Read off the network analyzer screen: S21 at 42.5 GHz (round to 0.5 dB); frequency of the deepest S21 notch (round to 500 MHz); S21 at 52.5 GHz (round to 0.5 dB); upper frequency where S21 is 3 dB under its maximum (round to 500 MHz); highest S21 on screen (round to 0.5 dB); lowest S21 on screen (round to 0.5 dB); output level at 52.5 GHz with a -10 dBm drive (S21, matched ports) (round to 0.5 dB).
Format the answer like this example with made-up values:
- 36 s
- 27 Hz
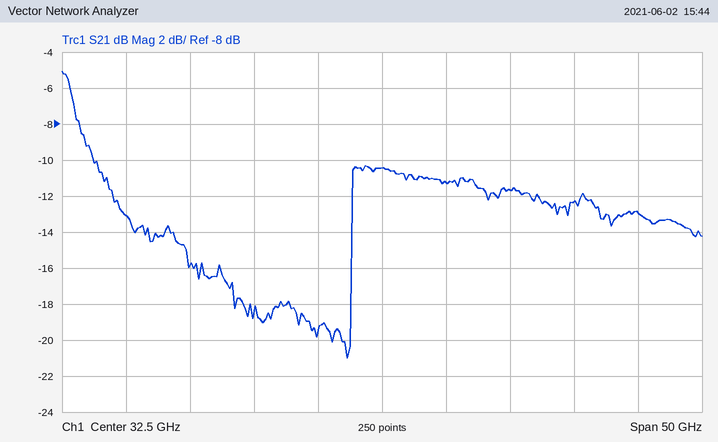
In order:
- -11.5 dB
- 30.0 GHz
- -13.0 dB
- 9.0 GHz
- -5.0 dB
- -21.0 dB
- -23.0 dBm
